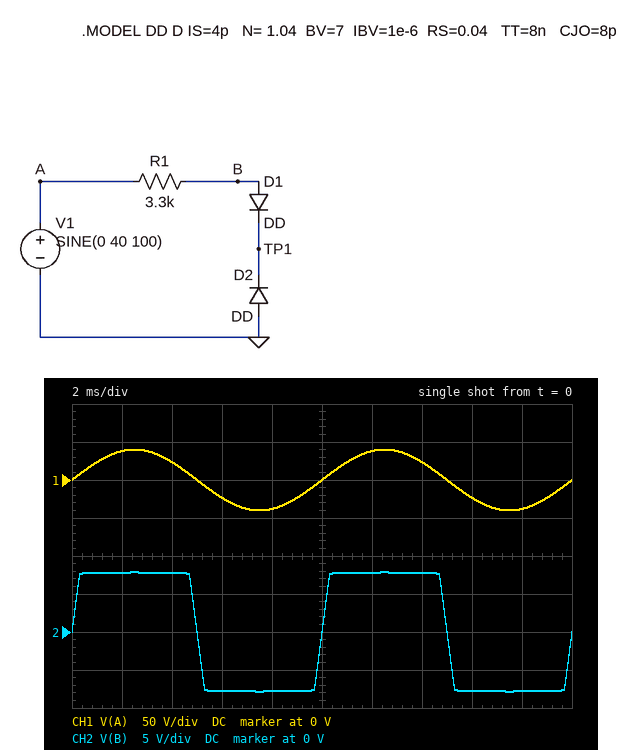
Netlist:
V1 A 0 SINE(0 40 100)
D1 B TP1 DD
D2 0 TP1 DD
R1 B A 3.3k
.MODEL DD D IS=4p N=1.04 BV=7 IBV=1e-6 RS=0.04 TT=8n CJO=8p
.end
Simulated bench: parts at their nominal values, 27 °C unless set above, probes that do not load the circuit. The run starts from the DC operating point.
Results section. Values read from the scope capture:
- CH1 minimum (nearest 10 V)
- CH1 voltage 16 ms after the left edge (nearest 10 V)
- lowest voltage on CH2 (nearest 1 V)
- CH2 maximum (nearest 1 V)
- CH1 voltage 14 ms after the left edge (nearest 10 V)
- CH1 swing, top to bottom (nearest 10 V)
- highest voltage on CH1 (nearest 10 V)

-40 V
-20 V
-8 V
8 V
20 V
80 V
40 V
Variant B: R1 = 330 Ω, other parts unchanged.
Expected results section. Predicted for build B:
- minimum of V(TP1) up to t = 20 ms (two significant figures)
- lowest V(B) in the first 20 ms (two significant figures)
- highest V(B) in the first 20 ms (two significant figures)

-650 mV
-8.0 V
8.0 V
